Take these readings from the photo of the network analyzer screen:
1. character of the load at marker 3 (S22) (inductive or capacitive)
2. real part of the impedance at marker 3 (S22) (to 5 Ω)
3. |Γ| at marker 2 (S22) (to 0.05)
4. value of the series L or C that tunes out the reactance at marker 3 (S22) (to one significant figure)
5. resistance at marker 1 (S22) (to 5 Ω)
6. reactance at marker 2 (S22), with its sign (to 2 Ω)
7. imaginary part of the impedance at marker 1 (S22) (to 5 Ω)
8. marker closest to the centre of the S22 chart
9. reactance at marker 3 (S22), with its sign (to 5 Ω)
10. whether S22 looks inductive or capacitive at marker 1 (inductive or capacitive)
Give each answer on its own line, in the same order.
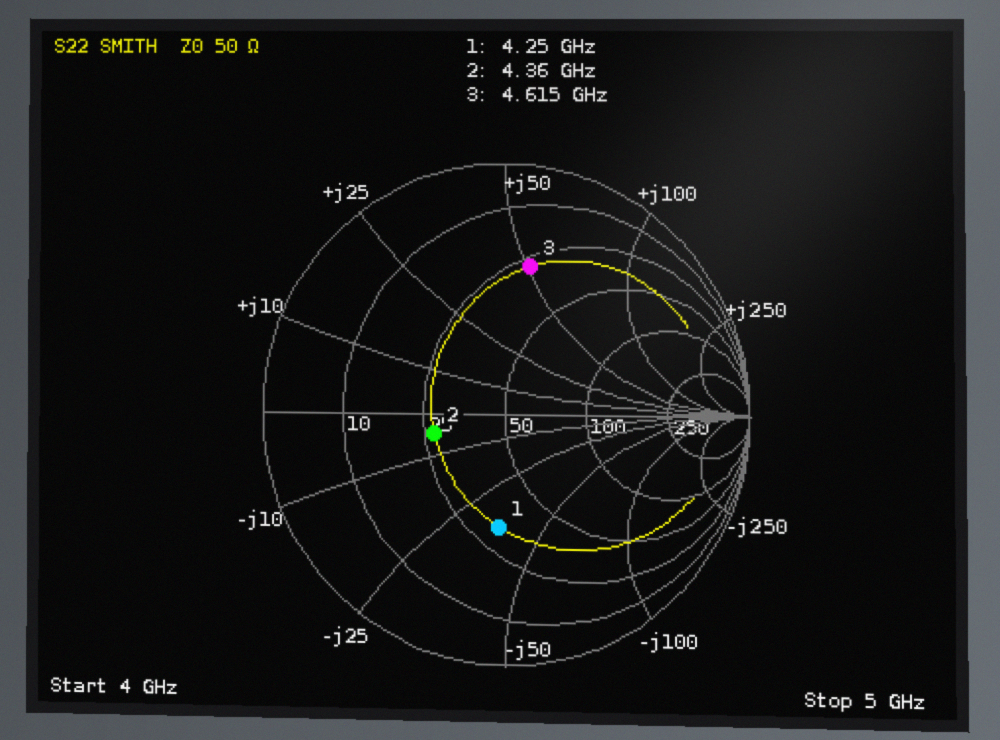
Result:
inductive
30 Ω
0.30
700 fF
30 Ω
-4 Ω
-35 Ω
marker 2
+50 Ω
capacitive
